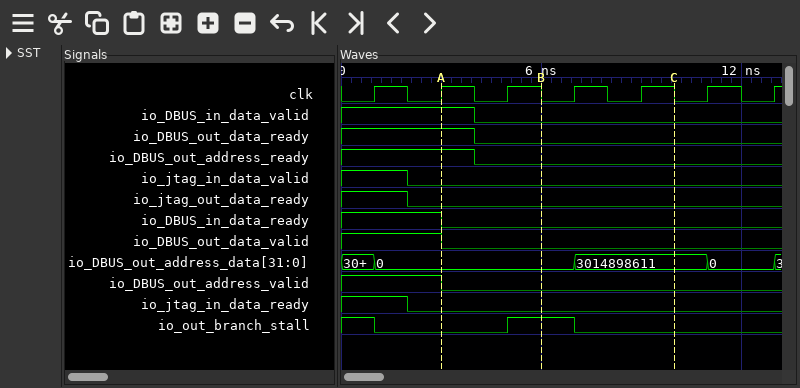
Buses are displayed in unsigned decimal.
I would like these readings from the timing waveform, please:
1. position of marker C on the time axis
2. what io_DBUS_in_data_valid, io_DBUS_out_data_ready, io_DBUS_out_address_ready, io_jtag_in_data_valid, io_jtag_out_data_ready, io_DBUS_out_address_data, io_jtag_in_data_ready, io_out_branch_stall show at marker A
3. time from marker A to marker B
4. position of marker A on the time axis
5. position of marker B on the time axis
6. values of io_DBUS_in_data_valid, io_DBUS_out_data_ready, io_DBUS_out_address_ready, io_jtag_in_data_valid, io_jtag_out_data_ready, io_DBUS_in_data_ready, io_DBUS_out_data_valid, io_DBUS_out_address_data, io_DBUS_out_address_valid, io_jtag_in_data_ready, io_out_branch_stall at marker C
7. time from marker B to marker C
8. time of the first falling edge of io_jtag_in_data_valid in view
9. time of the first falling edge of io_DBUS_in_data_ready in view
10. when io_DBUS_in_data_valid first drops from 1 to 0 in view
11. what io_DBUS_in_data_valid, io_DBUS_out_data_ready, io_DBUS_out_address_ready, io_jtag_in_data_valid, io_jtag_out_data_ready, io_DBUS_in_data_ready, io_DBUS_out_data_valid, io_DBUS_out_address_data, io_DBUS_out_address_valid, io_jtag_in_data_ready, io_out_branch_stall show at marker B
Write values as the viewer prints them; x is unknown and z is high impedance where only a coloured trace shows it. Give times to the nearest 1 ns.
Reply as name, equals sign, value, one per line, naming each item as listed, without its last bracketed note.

position of marker C on the time axis = 10 ns
what io_DBUS_in_data_valid, io_DBUS_out_data_ready, io_DBUS_out_address_ready, io_jtag_in_data_valid, io_jtag_out_data_ready, io_DBUS_out_address_data, io_jtag_in_data_ready, io_out_branch_stall show at marker A = io_DBUS_in_data_valid=1, io_DBUS_out_data_ready=1, io_DBUS_out_address_ready=1, io_jtag_in_data_valid=0, io_jtag_out_data_ready=0, io_DBUS_out_address_data=0, io_jtag_in_data_ready=0, io_out_branch_stall=0
time from marker A to marker B = 3 ns
position of marker A on the time axis = 3 ns
position of marker B on the time axis = 6 ns
values of io_DBUS_in_data_valid, io_DBUS_out_data_ready, io_DBUS_out_address_ready, io_jtag_in_data_valid, io_jtag_out_data_ready, io_DBUS_in_data_ready, io_DBUS_out_data_valid, io_DBUS_out_address_data, io_DBUS_out_address_valid, io_jtag_in_data_ready, io_out_branch_stall at marker C = io_DBUS_in_data_valid=0, io_DBUS_out_data_ready=0, io_DBUS_out_address_ready=0, io_jtag_in_data_valid=0, io_jtag_out_data_ready=0, io_DBUS_in_data_ready=0, io_DBUS_out_data_valid=0, io_DBUS_out_address_data=3014898611, io_DBUS_out_address_valid=0, io_jtag_in_data_ready=0, io_out_branch_stall=0
time from marker B to marker C = 4 ns
time of the first falling edge of io_jtag_in_data_valid in view = 2 ns
time of the first falling edge of io_DBUS_in_data_ready in view = 3 ns
when io_DBUS_in_data_valid first drops from 1 to 0 in view = 4 ns
what io_DBUS_in_data_valid, io_DBUS_out_data_ready, io_DBUS_out_address_ready, io_jtag_in_data_valid, io_jtag_out_data_ready, io_DBUS_in_data_ready, io_DBUS_out_data_valid, io_DBUS_out_address_data, io_DBUS_out_address_valid, io_jtag_in_data_ready, io_out_branch_stall show at marker B = io_DBUS_in_data_valid=0, io_DBUS_out_data_ready=0, io_DBUS_out_address_ready=0, io_jtag_in_data_valid=0, io_jtag_out_data_ready=0, io_DBUS_in_data_ready=0, io_DBUS_out_data_valid=0, io_DBUS_out_address_data=0, io_DBUS_out_address_valid=0, io_jtag_in_data_ready=0, io_out_branch_stall=1
